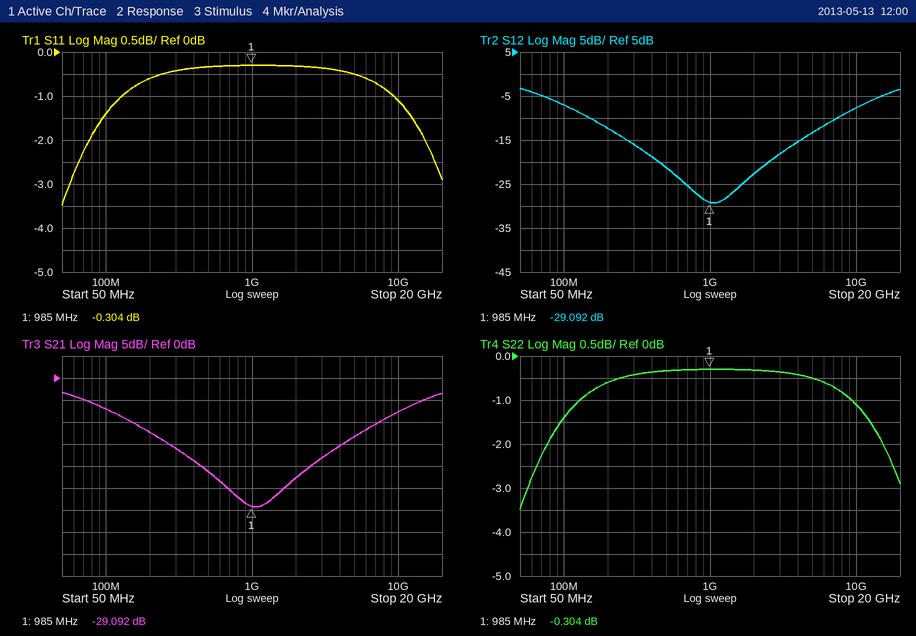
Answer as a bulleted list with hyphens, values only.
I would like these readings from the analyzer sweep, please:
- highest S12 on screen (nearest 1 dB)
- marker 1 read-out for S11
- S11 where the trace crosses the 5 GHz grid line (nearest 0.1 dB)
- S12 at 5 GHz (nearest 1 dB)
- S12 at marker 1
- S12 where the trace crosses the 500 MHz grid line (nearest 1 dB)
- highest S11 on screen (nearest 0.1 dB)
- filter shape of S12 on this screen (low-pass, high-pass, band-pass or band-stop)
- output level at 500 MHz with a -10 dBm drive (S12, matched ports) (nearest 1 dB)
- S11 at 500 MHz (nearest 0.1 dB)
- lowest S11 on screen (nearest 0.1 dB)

- -3 dB
- -0.304 dB
- -0.5 dB
- -13 dB
- -29.092 dB
- -21 dB
- -0.3 dB
- band-stop
- -31 dBm
- -0.3 dB
- -3.5 dB
